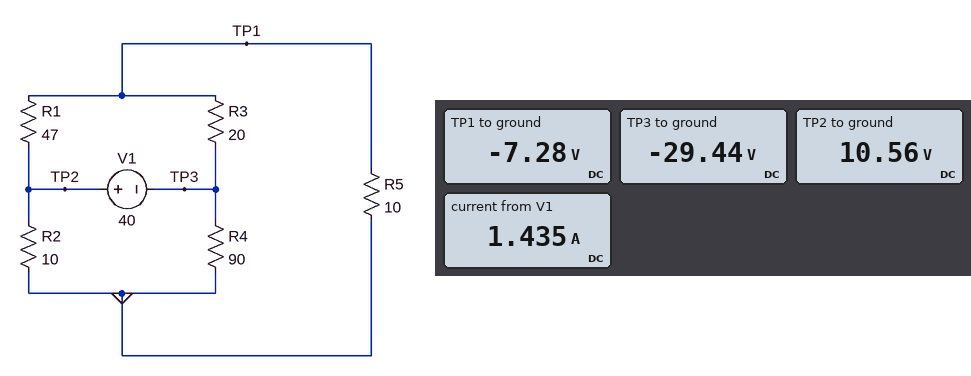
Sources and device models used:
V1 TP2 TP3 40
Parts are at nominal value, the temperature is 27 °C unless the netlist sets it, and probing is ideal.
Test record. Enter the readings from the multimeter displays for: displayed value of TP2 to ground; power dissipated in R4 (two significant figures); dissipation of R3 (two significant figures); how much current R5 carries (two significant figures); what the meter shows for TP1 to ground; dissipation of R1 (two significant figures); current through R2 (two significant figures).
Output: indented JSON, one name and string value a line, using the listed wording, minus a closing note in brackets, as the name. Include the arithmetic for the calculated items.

{
  "displayed value of TP2 to ground": "10.56 V",
  "power dissipated in R4": "(0 V - (-29.44 V))^2 / 90 Ω = 9.6 W",
  "dissipation of R3": "(-7.28 V - (-29.44 V))^2 / 20 Ω = 25 W",
  "how much current R5 carries": "(0 V - (-7.28 V)) / 10 Ω = 730 mA",
  "what the meter shows for TP1 to ground": "-7.28 V",
  "dissipation of R1": "(10.56 V - (-7.28 V))^2 / 47 Ω = 6.8 W",
  "current through R2": "(10.56 V) / 10 Ω = 1.1 A"
}
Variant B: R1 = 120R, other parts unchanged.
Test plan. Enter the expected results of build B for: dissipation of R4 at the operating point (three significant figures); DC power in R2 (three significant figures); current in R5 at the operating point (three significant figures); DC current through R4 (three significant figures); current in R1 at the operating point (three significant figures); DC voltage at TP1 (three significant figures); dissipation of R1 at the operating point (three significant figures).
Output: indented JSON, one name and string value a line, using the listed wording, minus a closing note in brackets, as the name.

{
  "dissipation of R4 at the operating point": "9.00 W",
  "DC power in R2": "13.3 W",
  "current in R5 at the operating point": "838 mA",
  "DC current through R4": "316 mA",
  "current in R1 at the operating point": "166 mA",
  "DC voltage at TP1": "-8.38 V",
  "dissipation of R1 at the operating point": "3.31 W"
}
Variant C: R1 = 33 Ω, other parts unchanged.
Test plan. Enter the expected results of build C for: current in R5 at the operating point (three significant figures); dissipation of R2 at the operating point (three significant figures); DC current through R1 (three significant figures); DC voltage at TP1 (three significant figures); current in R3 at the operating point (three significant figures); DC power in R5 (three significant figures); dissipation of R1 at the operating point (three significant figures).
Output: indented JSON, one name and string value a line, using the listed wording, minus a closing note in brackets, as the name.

{
  "current in R5 at the operating point": "665 mA",
  "dissipation of R2 at the operating point": "9.96 W",
  "DC current through R1": "504 mA",
  "DC voltage at TP1": "-6.65 V",
  "current in R3 at the operating point": "1.17 A",
  "DC power in R5": "4.42 W",
  "dissipation of R1 at the operating point": "8.38 W"
}
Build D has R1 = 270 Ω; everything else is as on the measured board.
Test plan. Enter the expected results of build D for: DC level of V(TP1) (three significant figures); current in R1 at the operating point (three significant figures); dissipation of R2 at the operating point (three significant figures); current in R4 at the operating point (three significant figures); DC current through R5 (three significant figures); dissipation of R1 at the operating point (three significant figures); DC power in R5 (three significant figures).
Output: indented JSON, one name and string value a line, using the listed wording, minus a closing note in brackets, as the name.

{
  "DC level of V(TP1)": "-8.84 V",
  "current in R1 at the operating point": "77.0 mA",
  "dissipation of R2 at the operating point": "14.3 W",
  "current in R4 at the operating point": "312 mA",
  "DC current through R5": "884 mA",
  "dissipation of R1 at the operating point": "1.60 W",
  "DC power in R5": "7.81 W"
}
